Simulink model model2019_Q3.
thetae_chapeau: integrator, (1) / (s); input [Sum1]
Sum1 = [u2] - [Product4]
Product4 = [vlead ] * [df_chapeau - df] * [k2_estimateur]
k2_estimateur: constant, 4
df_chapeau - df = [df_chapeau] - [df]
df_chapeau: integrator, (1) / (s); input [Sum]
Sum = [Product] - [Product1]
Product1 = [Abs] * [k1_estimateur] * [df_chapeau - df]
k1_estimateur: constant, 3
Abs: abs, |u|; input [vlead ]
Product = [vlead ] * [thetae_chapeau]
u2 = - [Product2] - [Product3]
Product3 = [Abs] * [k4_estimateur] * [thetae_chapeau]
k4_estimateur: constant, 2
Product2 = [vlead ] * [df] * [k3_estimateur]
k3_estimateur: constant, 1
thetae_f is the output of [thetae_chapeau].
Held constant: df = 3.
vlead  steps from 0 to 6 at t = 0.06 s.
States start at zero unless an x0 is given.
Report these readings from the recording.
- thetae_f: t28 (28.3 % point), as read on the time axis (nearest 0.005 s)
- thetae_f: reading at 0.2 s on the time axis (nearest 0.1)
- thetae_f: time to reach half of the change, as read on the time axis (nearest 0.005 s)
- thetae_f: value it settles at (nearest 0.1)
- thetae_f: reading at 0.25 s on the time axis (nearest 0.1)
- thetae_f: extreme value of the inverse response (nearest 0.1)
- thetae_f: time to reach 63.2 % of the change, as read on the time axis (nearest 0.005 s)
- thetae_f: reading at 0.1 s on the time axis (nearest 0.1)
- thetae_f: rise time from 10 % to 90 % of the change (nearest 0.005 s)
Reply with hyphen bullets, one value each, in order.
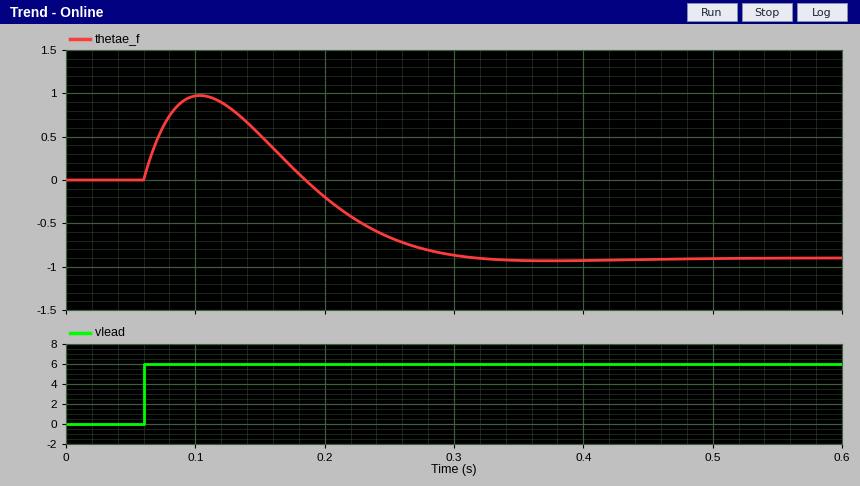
- 0.205 s
- -0.2
- 0.225 s
- -0.9
- -0.7
- 1.0
- 0.235 s
- 1.0
- 0.090 s
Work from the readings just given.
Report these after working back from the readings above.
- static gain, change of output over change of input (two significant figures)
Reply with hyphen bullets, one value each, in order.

- -0.15
